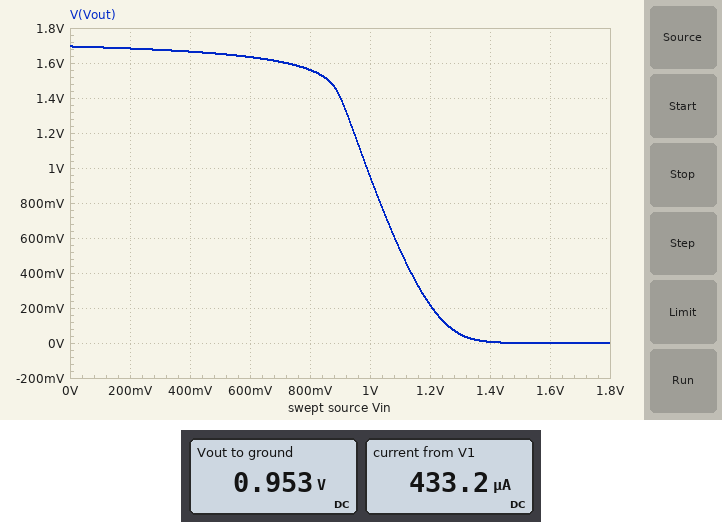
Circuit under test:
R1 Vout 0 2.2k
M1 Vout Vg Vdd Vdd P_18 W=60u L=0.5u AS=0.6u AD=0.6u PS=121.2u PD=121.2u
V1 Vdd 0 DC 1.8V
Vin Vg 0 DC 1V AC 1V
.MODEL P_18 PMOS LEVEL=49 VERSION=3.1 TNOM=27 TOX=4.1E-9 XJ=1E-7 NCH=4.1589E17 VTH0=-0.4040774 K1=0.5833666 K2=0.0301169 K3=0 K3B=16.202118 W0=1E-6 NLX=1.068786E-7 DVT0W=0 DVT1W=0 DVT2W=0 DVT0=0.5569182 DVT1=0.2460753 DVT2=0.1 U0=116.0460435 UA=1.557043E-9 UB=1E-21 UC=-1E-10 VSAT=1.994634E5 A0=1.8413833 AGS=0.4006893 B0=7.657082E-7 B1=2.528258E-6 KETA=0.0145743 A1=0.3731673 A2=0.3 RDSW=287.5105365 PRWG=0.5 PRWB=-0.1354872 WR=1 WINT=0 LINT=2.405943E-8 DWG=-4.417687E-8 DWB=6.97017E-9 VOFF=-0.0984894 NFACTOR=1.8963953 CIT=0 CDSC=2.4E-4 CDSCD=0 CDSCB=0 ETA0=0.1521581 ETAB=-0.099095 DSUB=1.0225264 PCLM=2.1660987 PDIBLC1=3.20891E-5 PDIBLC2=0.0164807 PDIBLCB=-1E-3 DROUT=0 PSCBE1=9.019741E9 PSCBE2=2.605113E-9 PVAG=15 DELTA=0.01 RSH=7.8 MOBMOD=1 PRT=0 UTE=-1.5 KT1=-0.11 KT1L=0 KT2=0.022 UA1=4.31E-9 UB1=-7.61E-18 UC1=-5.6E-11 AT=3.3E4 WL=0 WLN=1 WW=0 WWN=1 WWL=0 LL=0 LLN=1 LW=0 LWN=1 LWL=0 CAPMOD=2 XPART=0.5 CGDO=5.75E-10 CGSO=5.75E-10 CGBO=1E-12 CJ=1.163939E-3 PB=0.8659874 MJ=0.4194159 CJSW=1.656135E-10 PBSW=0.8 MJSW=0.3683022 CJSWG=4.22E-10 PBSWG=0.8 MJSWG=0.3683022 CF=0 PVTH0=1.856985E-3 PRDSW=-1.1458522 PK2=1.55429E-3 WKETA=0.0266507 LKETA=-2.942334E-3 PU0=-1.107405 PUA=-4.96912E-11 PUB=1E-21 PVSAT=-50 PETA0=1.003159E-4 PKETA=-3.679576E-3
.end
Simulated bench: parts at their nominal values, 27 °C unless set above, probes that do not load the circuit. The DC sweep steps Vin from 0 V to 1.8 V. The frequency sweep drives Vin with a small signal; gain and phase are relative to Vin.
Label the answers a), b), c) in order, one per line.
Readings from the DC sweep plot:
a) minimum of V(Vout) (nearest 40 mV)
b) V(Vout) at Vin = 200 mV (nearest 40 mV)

a) 0 V
b) 1.68 V
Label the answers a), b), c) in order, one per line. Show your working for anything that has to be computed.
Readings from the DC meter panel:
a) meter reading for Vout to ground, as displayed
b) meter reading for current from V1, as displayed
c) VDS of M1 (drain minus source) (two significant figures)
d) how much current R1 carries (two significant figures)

a) 0.953 V
b) 433.2 µA
c) 953 mV - 1.8 V = -850 mV
d) (953 mV) / 2.2 kΩ = 430 µA
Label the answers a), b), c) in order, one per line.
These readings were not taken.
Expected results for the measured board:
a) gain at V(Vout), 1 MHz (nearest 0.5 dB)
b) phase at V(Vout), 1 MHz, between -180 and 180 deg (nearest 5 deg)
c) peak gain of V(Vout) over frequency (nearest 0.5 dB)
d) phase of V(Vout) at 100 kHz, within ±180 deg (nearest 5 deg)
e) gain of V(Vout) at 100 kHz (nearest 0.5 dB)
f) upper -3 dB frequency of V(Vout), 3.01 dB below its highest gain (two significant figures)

a) -3.5 dB
b) 100 deg
c) 13.0 dB
d) 145 deg
e) 11.5 dB
f) 150 kHz
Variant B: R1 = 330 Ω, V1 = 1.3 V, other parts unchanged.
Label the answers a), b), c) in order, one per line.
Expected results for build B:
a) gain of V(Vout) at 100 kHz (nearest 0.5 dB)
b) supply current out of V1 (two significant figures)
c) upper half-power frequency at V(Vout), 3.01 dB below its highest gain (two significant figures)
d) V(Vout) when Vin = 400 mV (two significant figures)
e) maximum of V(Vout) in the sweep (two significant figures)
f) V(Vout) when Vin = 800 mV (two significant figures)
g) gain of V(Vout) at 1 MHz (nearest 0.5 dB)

a) -54.0 dB
b) 250 nA
c) 990 kHz
d) 230 mV
e) 650 mV
f) 7.2 mV
g) -57.0 dB
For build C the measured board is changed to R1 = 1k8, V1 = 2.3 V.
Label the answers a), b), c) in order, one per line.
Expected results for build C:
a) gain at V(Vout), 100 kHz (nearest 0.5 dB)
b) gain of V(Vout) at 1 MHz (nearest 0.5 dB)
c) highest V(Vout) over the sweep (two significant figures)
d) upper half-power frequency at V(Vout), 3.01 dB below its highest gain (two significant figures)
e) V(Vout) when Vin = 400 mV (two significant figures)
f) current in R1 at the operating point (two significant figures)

a) -10.5 dB
b) -13.0 dB
c) 2.2 V
d) 1.1 MHz
e) 2.1 V
f) 1.1 mA
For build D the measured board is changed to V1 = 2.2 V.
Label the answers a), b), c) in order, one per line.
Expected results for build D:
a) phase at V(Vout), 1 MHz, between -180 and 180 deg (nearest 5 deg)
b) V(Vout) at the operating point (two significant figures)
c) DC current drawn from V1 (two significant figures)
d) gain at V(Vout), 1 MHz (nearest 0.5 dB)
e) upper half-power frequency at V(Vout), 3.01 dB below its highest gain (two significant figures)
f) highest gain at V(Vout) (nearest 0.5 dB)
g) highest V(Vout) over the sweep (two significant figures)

a) 135 deg
b) 2.0 V
c) 900 µA
d) -13.5 dB
e) 980 kHz
f) -10.5 dB
g) 2.1 V
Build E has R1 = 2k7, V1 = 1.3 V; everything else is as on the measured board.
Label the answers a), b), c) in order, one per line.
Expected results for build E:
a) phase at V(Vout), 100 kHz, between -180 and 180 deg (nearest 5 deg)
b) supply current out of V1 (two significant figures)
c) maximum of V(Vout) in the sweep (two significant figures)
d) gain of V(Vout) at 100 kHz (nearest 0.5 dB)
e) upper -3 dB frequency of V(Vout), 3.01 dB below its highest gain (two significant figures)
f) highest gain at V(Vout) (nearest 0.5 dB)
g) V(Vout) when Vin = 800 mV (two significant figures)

a) 140 deg
b) 250 nA
c) 1.2 V
d) -37.5 dB
e) 120 kHz
f) -35.5 dB
g) 58 mV
